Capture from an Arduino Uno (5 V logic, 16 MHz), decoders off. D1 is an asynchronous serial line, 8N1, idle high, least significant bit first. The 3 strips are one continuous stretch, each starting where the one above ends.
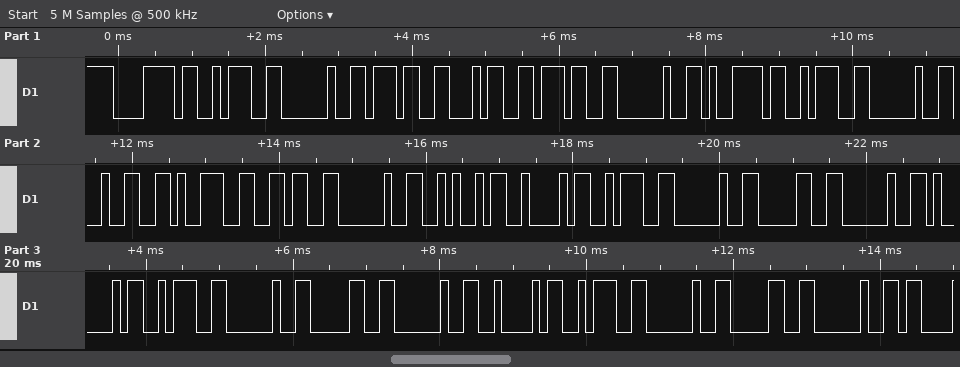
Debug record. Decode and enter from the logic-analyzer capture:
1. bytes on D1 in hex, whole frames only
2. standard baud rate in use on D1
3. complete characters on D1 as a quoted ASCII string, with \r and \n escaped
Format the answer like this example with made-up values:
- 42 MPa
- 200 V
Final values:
- 0x78 0x3A 0x20 0x37 0x34 0x37 0x20 0x79 0x3A 0x20 0x32 0x39 0x36 0x20 0x4A 0x42 0x3A 0x20 0x30 0x20 0x41 0x3A 0x20 0x30 0x20 0x42 0x3A 0x20 0x30 0x20
- 9600 baud
- "x: 747 y: 296 JB: 0 A: 0 B: 0 "
